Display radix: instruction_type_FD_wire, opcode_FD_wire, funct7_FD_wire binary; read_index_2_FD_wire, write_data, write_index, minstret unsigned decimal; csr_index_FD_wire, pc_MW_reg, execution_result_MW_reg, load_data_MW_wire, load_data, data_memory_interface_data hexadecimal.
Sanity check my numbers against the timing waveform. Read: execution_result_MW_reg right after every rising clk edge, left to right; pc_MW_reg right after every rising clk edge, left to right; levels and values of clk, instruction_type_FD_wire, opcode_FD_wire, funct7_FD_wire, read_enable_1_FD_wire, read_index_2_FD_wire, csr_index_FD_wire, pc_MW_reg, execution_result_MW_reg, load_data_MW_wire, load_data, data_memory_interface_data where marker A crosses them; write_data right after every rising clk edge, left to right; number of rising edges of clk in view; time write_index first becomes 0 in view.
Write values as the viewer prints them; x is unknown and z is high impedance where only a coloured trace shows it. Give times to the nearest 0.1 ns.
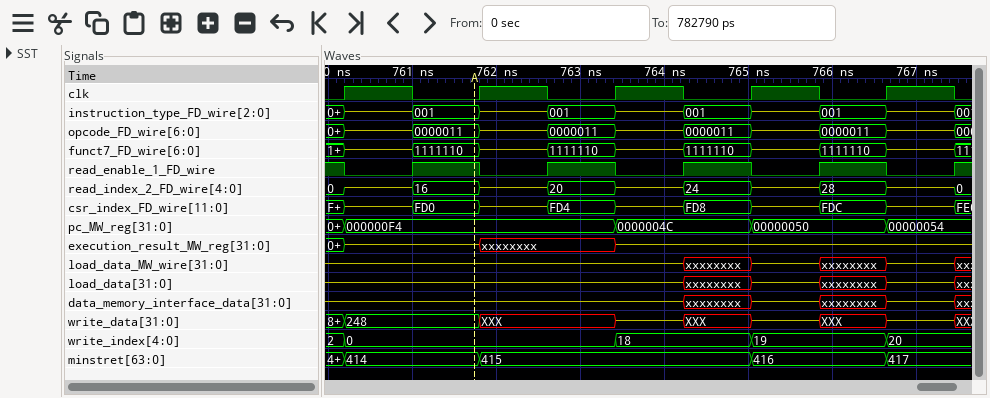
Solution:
z, xxxxxxxx, z, z, z
000000F4, 000000F4, 0000004C, 00000050, 00000054
clk=0, instruction_type_FD_wire=001, opcode_FD_wire=0000011, funct7_FD_wire=1111110, read_enable_1_FD_wire=1, read_index_2_FD_wire=16, csr_index_FD_wire=FD0, pc_MW_reg=000000F4, execution_result_MW_reg=z, load_data_MW_wire=z, load_data=z, data_memory_interface_data=z
248, XXX, z, z, z
5
760.2 ns
